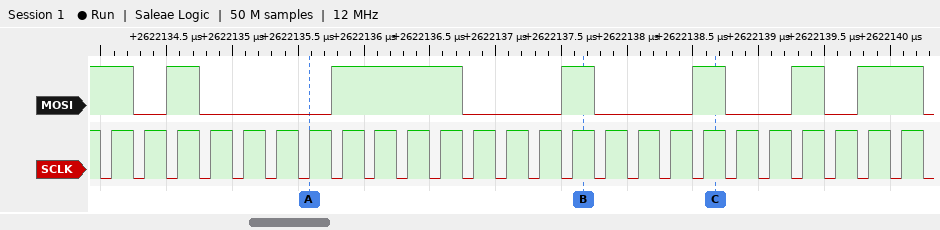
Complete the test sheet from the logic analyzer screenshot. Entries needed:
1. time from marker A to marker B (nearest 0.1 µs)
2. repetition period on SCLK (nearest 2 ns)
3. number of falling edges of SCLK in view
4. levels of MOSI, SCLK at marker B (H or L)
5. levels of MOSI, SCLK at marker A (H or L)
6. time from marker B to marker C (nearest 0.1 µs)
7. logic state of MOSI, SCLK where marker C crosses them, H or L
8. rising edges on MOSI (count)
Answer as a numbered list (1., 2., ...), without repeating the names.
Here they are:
1. 2.1 µs
2. 250 ns
3. 26
4. MOSI=H, SCLK=H
5. MOSI=L, SCLK=H
6. 1 µs
7. MOSI=H, SCLK=H
8. 6
